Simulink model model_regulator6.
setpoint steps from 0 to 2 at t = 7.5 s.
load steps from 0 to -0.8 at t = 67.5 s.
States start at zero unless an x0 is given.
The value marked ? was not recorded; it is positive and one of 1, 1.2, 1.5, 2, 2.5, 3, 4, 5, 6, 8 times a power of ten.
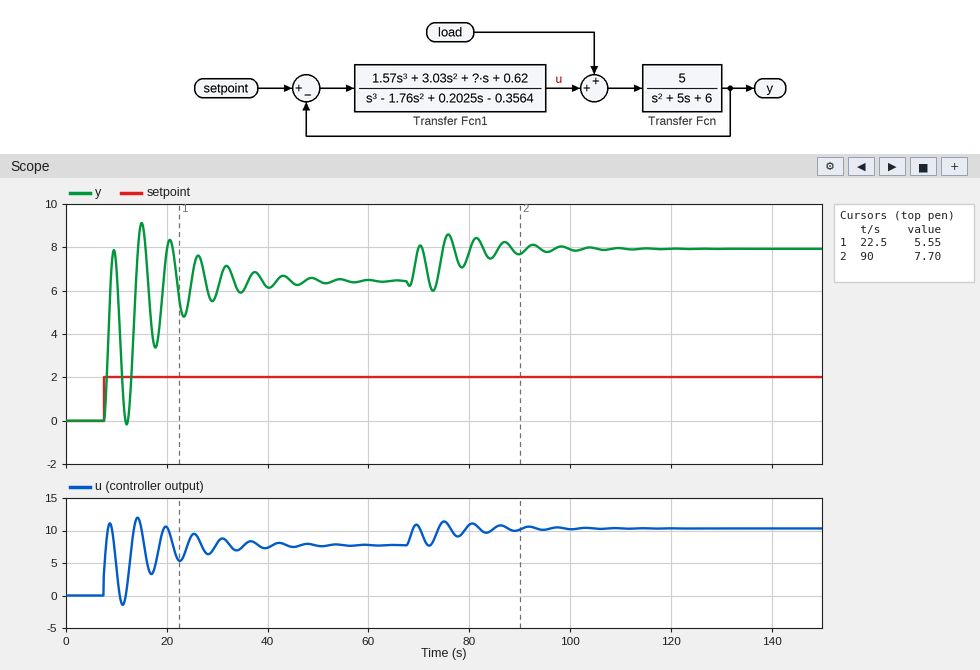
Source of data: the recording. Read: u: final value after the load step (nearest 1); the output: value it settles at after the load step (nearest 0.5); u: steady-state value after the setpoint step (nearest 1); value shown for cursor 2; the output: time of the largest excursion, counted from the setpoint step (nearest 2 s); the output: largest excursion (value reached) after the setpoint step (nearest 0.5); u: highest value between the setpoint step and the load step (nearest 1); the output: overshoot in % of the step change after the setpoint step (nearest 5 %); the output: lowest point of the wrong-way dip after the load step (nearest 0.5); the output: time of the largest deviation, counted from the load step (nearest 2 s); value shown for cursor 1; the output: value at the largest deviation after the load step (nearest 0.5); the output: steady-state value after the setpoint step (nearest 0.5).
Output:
10
8.0
8
7.70
8 s
9.0
12
40 %
6.0
8 s
5.55
8.5
6.5
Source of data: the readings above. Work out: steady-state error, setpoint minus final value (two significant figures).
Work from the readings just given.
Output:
-4.5
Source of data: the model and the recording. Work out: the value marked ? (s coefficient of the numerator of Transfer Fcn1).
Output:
1
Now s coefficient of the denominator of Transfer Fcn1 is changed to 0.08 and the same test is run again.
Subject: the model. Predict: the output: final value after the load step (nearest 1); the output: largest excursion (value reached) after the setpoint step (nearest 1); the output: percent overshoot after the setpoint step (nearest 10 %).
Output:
8
10
50 %
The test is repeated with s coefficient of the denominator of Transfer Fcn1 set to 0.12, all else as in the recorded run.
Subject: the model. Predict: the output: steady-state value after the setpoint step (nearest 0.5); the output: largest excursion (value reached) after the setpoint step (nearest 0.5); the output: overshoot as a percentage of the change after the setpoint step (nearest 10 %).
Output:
6.5
9.5
50 %
